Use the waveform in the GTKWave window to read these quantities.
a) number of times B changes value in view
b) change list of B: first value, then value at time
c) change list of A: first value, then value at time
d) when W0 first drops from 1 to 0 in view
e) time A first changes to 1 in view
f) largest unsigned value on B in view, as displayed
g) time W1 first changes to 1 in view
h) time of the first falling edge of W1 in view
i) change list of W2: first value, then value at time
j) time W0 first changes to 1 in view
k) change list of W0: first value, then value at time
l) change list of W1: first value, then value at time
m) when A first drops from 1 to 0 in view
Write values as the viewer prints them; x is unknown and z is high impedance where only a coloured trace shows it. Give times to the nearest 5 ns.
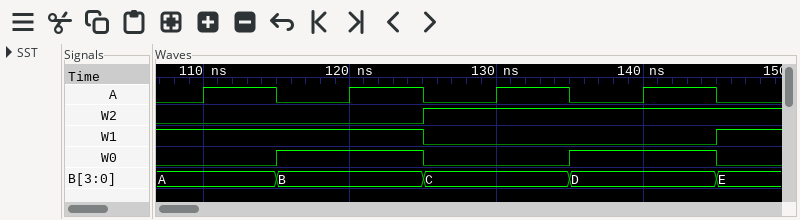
4
A, B at 115 ns, C at 125 ns, D at 135 ns, E at 145 ns
0, 1 at 110 ns, 0 at 115 ns, 1 at 120 ns, 0 at 125 ns, 1 at 130 ns, 0 at 135 ns, 1 at 140 ns, 0 at 145 ns
125 ns
110 ns
E
145 ns
125 ns
0, 1 at 125 ns
115 ns
0, 1 at 115 ns, 0 at 125 ns, 1 at 135 ns, 0 at 145 ns
1, 0 at 125 ns, 1 at 145 ns
115 ns
